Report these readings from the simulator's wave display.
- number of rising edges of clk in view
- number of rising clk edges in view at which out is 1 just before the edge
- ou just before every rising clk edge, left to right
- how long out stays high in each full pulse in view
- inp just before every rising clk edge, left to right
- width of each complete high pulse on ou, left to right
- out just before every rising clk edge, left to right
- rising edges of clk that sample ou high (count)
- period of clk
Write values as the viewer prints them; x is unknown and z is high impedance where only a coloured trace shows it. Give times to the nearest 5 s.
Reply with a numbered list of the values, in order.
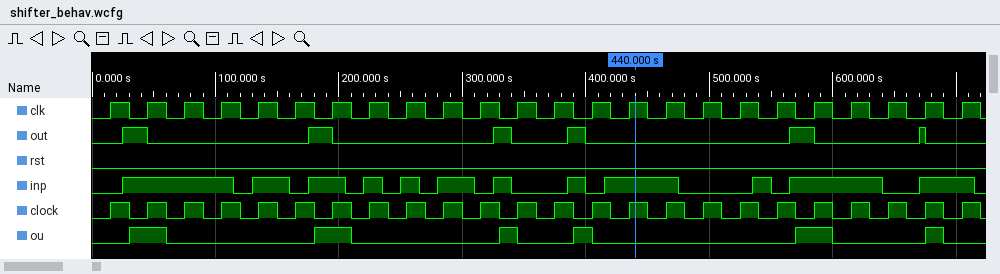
1. 24
2. 4
3. 0 1 0 0 0 0 1 0 0 0 0 1 0 1 0 0 0 0 0 1 0 0 0 0
4. 20 s, 20 s, 15 s, 15 s, 20 s, 5 s
5. 0 1 1 1 1 0 1 1 1 1 0 0 0 0 1 1 0 0 0 1 1 0 1 1
6. 30 s, 30 s, 15 s, 15 s, 30 s, 15 s
7. 0 1 0 0 0 0 1 0 0 0 0 0 0 0 0 0 0 0 0 1 0 0 1 0
8. 5
9. 30 s
